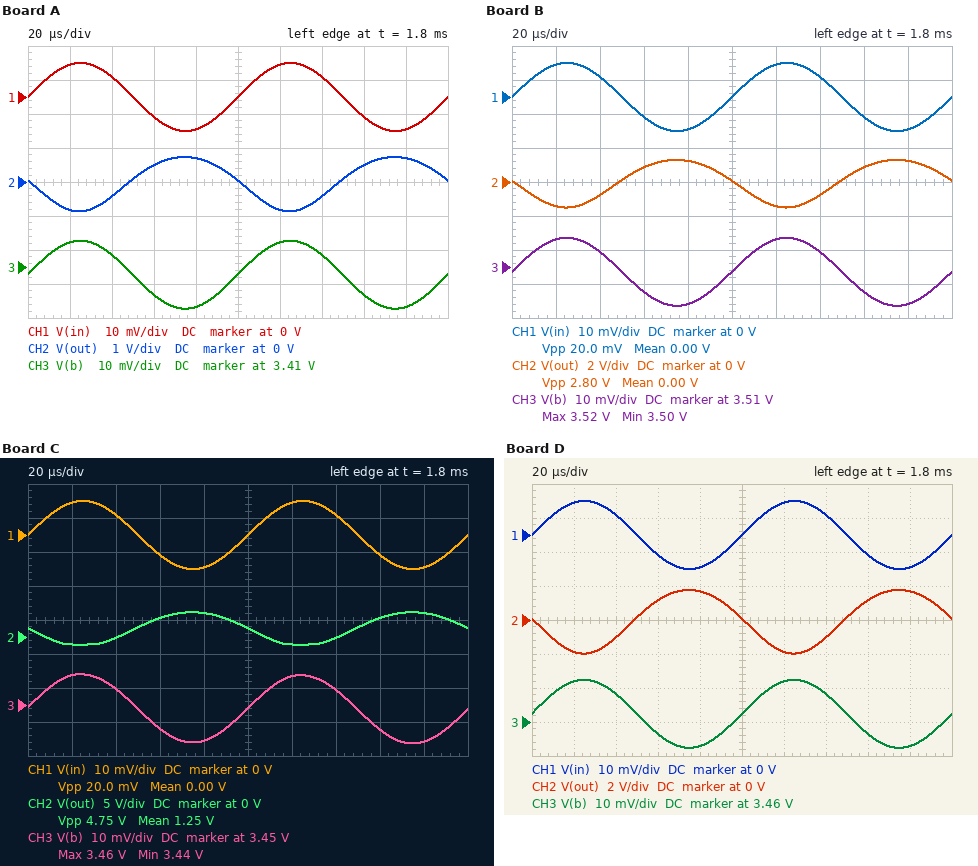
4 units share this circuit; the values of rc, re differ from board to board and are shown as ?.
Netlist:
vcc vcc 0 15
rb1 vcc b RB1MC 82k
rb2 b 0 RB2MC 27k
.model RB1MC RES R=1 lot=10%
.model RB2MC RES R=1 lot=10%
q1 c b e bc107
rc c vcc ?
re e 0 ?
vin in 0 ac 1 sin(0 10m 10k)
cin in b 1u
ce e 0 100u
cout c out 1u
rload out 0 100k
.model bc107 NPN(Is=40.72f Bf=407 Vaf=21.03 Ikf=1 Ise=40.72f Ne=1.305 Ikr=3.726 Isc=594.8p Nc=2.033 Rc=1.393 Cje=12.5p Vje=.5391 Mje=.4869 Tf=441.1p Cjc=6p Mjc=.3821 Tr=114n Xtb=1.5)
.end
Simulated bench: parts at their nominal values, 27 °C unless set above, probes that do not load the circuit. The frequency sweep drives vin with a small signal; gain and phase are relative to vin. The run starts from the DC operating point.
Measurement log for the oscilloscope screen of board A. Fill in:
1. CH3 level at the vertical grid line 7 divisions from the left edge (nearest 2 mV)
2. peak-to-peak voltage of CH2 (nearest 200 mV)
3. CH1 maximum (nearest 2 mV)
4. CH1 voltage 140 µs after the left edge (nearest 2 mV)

3.414 V
1.6 V
10 mV
6 mV
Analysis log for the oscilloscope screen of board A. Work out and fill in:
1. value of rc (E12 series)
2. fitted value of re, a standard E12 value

560 Ω
680 Ω
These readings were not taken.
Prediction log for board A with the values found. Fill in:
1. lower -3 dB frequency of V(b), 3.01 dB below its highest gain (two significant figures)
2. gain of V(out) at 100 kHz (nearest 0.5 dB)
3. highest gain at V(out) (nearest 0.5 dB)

21 Hz
38.0 dB
38.0 dB
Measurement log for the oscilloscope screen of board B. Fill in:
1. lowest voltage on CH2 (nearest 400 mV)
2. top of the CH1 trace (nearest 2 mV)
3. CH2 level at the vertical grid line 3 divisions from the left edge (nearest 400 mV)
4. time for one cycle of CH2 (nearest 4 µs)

-1.6 V
10 mV
800 mV
100 µs
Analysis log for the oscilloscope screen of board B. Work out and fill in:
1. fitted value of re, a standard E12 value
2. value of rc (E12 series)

1.2 kΩ
1.8 kΩ
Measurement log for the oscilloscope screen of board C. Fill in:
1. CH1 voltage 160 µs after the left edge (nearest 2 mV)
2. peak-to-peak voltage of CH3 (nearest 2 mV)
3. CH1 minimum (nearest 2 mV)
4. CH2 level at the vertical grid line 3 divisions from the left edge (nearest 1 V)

-6 mV
20 mV
-10 mV
3 V
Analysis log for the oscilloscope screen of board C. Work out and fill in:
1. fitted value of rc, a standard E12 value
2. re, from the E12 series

4.7 kΩ
1.2 kΩ
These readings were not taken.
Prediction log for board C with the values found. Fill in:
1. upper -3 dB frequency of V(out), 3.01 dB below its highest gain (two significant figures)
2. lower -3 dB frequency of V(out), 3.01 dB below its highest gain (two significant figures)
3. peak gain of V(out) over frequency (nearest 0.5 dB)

11 MHz
170 Hz
48.5 dB
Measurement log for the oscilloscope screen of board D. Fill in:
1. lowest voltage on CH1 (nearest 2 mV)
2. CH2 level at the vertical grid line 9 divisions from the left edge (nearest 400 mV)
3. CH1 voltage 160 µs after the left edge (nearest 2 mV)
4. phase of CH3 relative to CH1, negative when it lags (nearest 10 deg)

-10 mV
1.6 V
-6 mV
0 deg
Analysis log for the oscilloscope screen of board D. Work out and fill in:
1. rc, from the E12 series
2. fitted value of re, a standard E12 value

2.2 kΩ
1 kΩ
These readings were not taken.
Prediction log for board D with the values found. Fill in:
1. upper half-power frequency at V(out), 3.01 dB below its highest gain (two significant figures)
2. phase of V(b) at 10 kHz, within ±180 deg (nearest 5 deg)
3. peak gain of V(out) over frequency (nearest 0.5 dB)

34 MHz
0 deg
45.5 dB
